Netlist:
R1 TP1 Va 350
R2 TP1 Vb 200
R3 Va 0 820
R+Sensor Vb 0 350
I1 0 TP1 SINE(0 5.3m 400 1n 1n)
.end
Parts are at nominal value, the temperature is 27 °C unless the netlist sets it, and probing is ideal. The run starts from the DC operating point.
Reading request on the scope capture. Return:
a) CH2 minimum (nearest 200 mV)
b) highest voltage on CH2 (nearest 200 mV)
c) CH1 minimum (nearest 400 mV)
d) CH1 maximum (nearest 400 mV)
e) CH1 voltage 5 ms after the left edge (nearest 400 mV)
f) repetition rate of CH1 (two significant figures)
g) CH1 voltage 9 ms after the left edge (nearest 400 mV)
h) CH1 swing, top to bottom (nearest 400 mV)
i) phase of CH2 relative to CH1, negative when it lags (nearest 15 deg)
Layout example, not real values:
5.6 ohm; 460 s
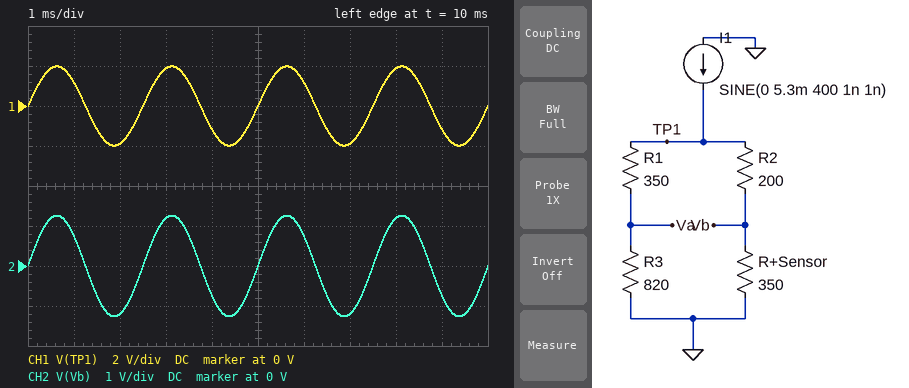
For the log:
-1.2 V; 1.2 V; -2.0 V; 2.0 V; 0 V; 400 Hz; -1.2 V; 4.0 V; 0 deg
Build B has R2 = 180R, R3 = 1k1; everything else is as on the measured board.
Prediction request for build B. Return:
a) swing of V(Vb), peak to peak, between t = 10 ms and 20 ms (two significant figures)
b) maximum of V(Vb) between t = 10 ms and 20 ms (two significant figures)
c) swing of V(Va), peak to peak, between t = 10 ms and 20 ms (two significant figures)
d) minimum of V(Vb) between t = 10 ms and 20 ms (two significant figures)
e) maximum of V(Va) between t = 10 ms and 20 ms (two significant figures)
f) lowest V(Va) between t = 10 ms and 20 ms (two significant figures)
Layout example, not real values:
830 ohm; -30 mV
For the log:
2.7 V; 1.4 V; 3.1 V; -1.4 V; 1.6 V; -1.6 V
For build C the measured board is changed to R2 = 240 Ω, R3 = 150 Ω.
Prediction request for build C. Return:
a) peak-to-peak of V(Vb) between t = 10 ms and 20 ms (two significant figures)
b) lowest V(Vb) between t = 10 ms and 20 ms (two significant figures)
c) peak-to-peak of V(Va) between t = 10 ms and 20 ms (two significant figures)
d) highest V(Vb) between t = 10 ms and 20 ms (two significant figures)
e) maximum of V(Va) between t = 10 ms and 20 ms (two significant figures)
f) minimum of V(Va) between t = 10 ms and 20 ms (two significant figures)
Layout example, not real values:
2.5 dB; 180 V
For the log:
1.7 V; -850 mV; 860 mV; 850 mV; 430 mV; -430 mV
